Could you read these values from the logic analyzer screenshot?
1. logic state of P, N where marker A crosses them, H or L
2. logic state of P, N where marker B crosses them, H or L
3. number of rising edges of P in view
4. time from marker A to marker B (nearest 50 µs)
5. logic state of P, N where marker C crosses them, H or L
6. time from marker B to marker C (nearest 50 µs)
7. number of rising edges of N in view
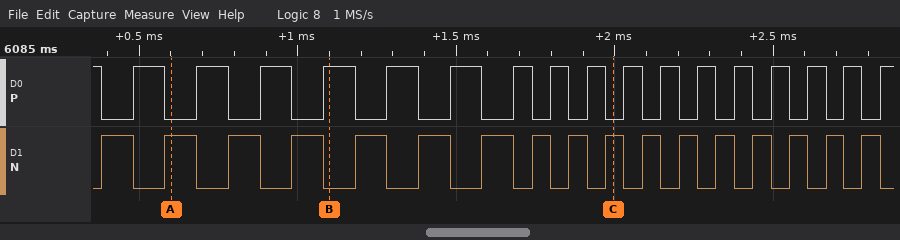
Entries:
P=L, N=H
P=H, N=L
17
500 µs
P=L, N=H
900 µs
17
